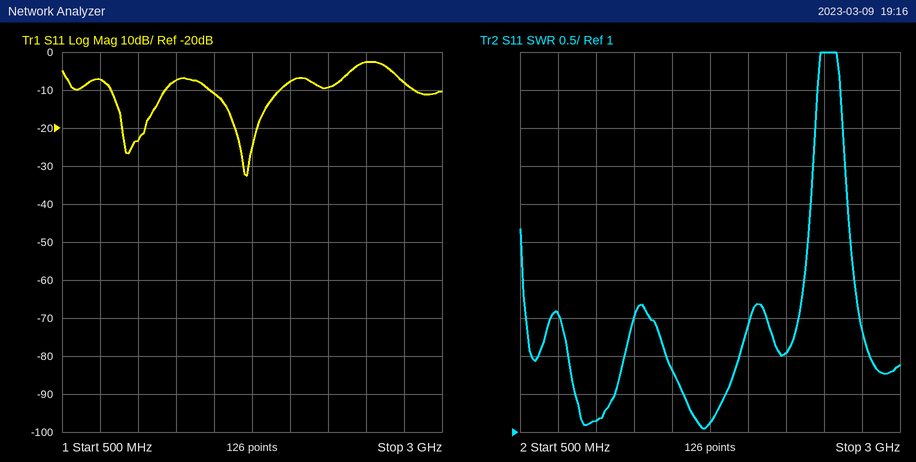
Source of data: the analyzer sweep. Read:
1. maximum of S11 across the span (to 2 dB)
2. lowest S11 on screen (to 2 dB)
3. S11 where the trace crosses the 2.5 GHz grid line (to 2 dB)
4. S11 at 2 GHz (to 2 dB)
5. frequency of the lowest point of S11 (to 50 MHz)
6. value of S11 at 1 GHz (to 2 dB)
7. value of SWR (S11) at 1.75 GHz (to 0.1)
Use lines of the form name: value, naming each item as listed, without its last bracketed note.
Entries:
maximum of S11 across the span: -2 dB
lowest S11 on screen: -32 dB
S11 where the trace crosses the 2.5 GHz grid line: -2 dB
S11 at 2 GHz: -8 dB
frequency of the lowest point of S11: 1.70 GHz
value of S11 at 1 GHz: -24 dB
value of SWR (S11) at 1.75 GHz: 1.1
